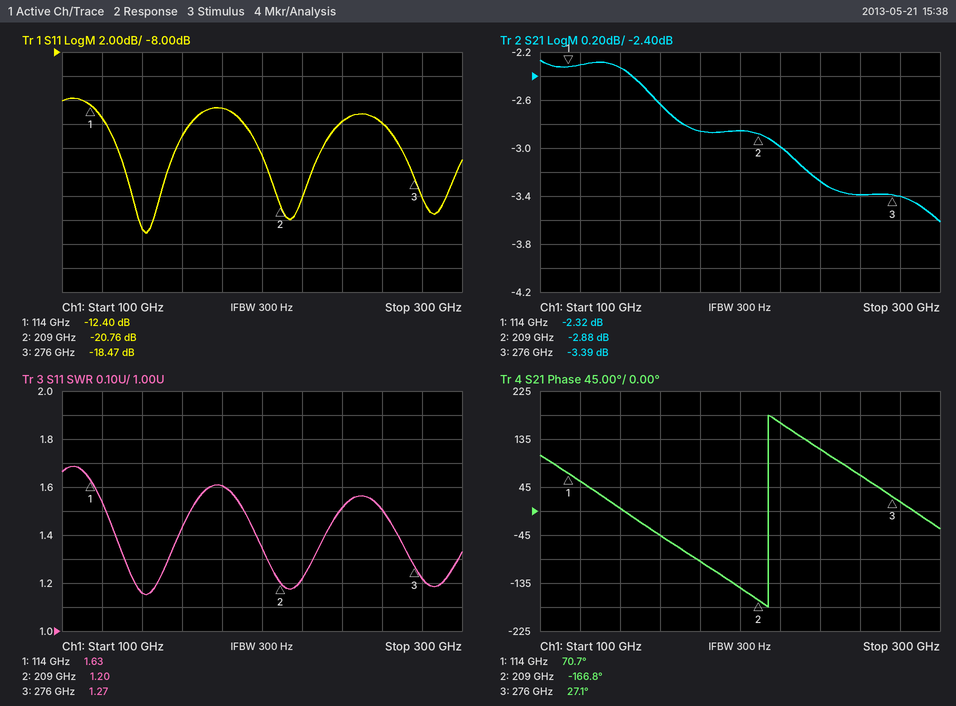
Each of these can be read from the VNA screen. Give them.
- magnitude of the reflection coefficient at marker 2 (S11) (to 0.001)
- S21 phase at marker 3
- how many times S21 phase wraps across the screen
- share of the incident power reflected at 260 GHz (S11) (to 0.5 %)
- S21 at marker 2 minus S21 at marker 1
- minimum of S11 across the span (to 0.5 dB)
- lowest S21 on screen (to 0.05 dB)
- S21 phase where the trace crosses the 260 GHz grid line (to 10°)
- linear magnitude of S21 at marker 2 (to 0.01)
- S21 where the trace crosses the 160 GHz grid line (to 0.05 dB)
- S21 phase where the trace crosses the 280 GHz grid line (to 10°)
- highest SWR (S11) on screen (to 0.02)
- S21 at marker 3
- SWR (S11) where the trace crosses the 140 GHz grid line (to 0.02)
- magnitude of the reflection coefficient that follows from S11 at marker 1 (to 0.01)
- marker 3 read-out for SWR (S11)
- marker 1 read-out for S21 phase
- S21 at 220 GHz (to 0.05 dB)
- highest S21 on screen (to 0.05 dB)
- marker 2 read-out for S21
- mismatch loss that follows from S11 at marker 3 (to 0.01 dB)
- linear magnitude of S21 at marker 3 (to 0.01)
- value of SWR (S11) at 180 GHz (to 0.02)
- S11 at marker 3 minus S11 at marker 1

0.092
27.1°
1
4.0 %
-0.56 dB
-23.0 dB
-3.60 dB
70°
0.72
-2.65 dB
20°
1.68
-3.39 dB
1.16
0.24
1.27
70.7°
-3.00 dB
-2.25 dB
-2.88 dB
0.06 dB
0.68
1.60
-6.07 dB
